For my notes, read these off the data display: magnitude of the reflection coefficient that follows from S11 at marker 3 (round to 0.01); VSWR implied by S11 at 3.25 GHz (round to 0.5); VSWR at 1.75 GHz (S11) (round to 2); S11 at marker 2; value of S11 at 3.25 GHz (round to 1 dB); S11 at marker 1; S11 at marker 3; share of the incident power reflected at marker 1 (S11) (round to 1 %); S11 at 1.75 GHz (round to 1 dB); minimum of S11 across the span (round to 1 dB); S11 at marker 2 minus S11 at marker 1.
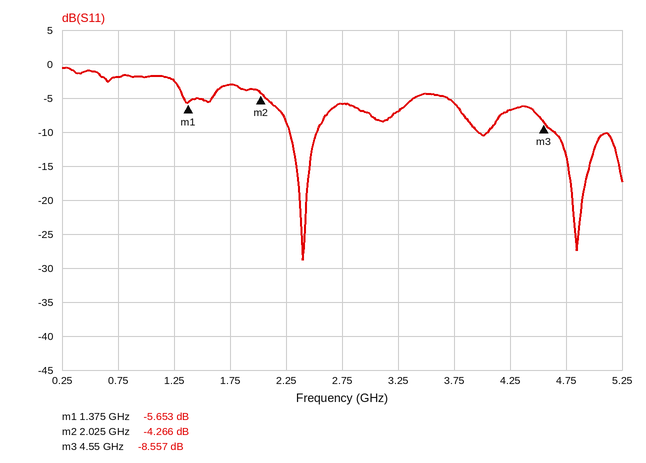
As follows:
0.37
2.5
6
-4.266 dB
-7 dB
-5.653 dB
-8.557 dB
27 %
-3 dB
-29 dB
1.387 dB
